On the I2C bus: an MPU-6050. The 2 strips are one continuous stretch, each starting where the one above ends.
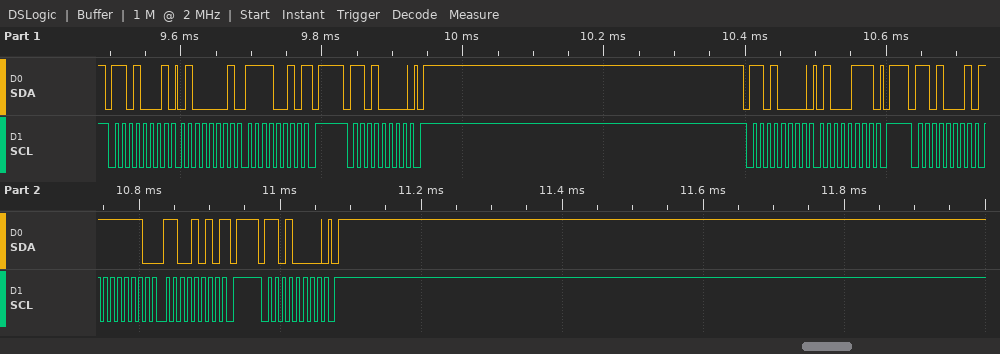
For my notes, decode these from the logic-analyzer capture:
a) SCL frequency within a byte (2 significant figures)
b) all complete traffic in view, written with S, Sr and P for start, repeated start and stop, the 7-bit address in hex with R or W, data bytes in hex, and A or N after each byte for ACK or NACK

100 kHz
S 68R A 41 A F2 N P S 68W A P S 68W A 47 A P S 68R A FE A CA N P S 68W A P
